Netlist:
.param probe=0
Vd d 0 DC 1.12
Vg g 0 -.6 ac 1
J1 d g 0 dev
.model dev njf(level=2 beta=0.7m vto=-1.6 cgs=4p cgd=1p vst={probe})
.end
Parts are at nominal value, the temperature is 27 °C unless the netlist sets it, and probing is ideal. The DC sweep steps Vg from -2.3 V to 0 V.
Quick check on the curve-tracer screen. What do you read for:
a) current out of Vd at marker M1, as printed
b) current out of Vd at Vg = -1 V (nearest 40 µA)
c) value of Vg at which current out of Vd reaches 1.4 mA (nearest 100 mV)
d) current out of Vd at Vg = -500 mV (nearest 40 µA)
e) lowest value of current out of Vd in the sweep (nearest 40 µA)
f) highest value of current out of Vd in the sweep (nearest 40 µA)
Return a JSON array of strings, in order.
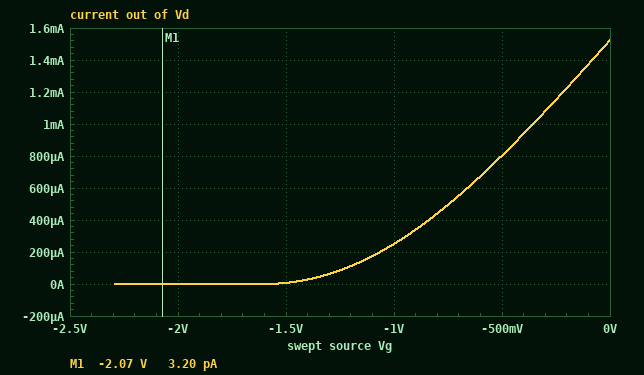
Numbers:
["3.20 pA", "240 µA", "-100 mV", "800 µA", "0 A", "1.52 mA"]
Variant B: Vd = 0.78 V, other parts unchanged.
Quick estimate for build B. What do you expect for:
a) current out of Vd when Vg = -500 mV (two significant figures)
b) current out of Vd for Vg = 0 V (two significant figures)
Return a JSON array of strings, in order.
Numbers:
["720 µA", "1.3 mA"]
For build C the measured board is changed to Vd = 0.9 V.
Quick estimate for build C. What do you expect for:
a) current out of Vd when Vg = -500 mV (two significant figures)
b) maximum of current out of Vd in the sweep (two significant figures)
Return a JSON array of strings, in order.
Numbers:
["760 µA", "1.4 mA"]
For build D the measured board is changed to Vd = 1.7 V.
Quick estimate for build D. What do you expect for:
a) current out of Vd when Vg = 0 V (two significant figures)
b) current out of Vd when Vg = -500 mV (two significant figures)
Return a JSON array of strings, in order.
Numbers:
["1.7 mA", "840 µA"]
